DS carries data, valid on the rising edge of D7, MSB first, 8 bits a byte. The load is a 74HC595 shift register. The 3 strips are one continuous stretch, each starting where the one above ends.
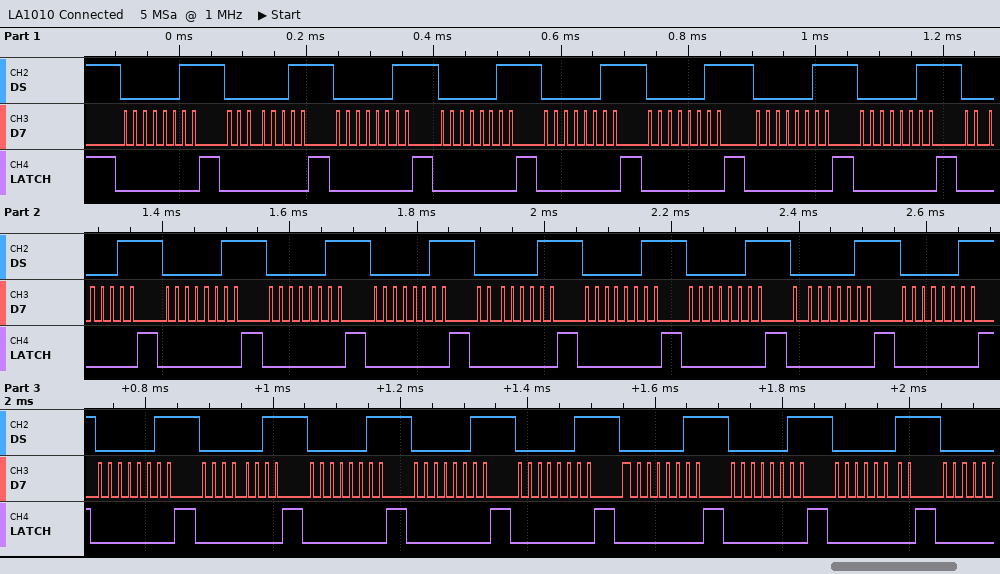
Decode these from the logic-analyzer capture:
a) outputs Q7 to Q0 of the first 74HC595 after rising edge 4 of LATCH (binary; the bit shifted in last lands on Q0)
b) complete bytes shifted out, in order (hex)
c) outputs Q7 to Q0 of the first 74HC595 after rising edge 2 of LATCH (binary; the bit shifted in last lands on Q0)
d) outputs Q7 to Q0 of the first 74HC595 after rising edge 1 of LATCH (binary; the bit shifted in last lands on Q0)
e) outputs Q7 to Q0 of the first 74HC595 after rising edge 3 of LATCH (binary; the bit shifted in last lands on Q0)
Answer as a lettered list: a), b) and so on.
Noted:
a) 00000011
b) 03 03 03 03 03 03 03 03 03 03 03 03 03 03 03 03 03 03 03 03 03 03 03 03 03
c) 00000011
d) 00000011
e) 00000011
